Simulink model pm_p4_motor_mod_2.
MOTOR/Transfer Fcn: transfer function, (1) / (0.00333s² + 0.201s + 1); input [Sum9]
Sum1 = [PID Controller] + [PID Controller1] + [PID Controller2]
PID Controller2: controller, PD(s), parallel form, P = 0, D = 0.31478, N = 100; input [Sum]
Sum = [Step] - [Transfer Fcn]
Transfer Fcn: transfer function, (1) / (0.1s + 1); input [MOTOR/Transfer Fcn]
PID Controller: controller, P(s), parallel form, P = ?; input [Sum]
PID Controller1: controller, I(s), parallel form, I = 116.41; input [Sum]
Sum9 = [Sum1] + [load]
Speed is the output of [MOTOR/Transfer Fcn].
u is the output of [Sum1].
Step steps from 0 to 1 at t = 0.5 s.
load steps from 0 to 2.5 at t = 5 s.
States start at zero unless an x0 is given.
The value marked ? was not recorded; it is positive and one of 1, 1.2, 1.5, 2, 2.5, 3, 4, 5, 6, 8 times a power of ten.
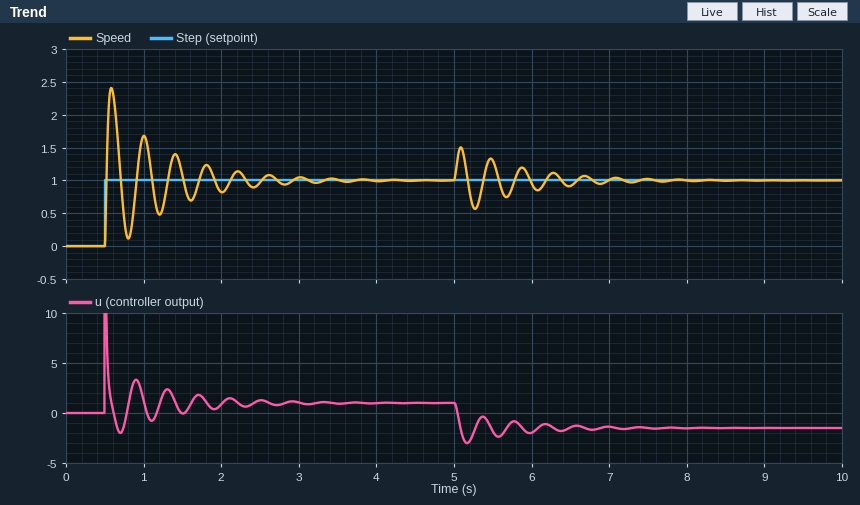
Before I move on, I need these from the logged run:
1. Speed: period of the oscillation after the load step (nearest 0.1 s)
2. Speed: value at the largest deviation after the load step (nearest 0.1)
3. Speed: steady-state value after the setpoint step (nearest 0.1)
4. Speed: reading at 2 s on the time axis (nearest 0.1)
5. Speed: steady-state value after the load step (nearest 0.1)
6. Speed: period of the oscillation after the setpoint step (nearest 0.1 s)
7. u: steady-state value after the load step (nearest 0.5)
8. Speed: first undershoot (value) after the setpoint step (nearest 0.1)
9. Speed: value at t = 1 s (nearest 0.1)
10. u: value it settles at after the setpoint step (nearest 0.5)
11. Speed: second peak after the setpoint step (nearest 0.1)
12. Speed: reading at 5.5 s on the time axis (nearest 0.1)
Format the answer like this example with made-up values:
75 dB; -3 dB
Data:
0.4 s; 1.5; 1.0; 0.8; 1.0; 0.4 s; -1.5; 0.1; 1.7; 1.0; 1.7; 1.3
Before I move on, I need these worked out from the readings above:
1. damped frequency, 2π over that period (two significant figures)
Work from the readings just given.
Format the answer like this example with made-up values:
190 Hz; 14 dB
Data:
16 rad/s
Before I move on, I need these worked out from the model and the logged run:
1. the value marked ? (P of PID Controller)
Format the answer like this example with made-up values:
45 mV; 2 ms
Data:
5
